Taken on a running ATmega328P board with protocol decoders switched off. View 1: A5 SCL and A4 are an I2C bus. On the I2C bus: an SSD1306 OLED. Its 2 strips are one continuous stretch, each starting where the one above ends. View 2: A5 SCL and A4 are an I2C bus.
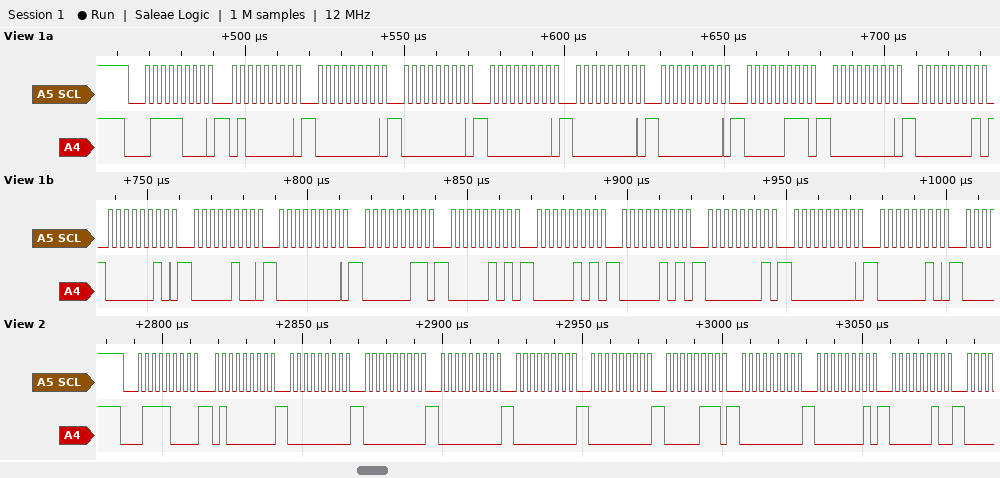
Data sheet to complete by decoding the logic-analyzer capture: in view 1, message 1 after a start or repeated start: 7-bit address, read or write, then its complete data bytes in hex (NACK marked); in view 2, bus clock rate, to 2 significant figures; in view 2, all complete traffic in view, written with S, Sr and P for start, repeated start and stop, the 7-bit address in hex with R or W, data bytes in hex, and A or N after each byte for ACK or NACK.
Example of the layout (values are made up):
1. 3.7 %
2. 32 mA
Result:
1. 0x3C write: 40 00 00 00 00 00 07 00 01 02 04 00 03 05 05 05 01 00 02
2. 400 kHz
3. S 3CW A 40 A 00 A 00 A 00 A 00 A 00 A 07 A 00 A 01 A 02 A
